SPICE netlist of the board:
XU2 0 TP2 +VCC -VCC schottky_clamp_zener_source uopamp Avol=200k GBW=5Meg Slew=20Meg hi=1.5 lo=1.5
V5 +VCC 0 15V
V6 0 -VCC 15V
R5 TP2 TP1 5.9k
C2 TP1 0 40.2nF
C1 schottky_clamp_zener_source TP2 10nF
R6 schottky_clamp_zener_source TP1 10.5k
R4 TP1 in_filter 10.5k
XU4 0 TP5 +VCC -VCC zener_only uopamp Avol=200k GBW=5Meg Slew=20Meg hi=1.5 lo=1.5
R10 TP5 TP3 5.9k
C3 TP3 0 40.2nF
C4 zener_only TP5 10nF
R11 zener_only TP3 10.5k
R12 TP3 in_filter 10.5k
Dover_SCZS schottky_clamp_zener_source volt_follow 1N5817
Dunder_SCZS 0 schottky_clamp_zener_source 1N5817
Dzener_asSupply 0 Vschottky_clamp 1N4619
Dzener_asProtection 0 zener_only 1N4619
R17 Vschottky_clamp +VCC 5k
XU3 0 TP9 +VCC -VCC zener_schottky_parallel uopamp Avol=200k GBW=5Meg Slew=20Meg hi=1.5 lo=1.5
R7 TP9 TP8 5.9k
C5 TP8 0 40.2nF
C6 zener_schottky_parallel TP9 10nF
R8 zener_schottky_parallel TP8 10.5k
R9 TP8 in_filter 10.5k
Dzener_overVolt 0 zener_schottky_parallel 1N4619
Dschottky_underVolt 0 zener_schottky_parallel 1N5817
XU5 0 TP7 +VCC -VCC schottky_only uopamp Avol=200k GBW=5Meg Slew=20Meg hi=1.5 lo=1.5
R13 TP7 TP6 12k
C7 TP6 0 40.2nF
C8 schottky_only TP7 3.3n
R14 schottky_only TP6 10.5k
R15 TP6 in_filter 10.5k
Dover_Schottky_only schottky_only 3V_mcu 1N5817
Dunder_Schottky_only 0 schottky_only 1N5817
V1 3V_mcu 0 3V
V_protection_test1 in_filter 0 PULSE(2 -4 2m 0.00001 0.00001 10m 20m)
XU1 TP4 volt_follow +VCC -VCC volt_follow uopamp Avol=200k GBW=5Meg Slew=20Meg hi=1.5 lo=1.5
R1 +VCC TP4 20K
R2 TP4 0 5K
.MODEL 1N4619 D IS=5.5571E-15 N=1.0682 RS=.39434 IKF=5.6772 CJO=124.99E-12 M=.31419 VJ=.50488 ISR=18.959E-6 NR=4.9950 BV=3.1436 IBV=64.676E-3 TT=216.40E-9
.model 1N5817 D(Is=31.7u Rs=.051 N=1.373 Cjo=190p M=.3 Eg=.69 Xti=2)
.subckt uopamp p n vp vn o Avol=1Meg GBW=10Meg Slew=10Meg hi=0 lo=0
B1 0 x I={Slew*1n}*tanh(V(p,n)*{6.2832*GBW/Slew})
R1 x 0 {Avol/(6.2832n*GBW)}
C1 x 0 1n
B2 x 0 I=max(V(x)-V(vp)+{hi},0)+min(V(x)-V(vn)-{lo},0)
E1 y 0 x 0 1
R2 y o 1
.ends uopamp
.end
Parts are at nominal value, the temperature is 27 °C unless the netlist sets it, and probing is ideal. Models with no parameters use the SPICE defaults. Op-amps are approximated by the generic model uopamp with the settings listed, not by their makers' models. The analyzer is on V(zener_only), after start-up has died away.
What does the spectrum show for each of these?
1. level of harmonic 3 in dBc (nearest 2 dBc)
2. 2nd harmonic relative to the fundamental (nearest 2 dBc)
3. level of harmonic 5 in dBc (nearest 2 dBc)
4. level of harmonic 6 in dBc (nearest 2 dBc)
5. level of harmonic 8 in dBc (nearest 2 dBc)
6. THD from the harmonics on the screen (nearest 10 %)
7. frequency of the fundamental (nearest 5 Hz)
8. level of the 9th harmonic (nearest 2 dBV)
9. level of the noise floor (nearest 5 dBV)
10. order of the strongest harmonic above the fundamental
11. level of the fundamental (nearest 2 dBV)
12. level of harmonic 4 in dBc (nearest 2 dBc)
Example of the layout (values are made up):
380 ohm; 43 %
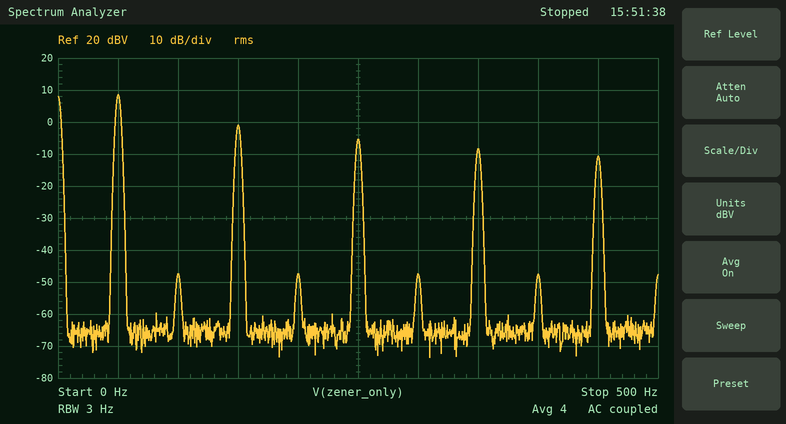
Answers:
-10 dBc; -56 dBc; -14 dBc; -56 dBc; -56 dBc; 40 %; 50 Hz; -10 dBV; -65 dBV; 3; 8 dBV; -56 dBc
